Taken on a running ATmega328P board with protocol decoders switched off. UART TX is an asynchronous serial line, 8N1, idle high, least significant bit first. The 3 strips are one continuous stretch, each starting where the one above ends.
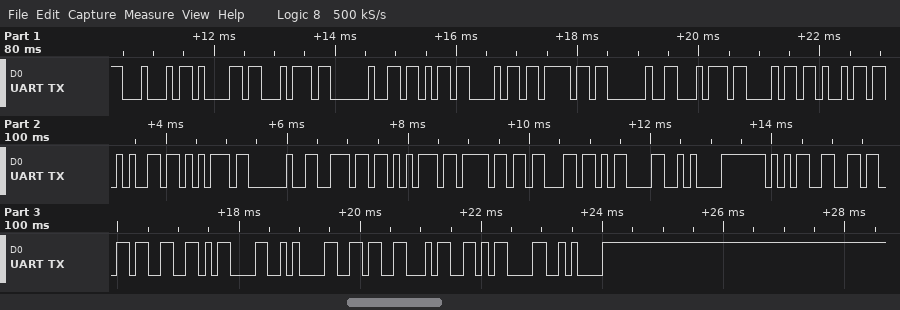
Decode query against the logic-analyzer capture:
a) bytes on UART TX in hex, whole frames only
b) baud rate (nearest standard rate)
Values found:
44 61 74 20 6B 68 6F 20 74 68 69 65 75 20 6E 75 6F 63 0D 0A 35 36 33 0D 0A 36 34 0D 0A
9600 baud
